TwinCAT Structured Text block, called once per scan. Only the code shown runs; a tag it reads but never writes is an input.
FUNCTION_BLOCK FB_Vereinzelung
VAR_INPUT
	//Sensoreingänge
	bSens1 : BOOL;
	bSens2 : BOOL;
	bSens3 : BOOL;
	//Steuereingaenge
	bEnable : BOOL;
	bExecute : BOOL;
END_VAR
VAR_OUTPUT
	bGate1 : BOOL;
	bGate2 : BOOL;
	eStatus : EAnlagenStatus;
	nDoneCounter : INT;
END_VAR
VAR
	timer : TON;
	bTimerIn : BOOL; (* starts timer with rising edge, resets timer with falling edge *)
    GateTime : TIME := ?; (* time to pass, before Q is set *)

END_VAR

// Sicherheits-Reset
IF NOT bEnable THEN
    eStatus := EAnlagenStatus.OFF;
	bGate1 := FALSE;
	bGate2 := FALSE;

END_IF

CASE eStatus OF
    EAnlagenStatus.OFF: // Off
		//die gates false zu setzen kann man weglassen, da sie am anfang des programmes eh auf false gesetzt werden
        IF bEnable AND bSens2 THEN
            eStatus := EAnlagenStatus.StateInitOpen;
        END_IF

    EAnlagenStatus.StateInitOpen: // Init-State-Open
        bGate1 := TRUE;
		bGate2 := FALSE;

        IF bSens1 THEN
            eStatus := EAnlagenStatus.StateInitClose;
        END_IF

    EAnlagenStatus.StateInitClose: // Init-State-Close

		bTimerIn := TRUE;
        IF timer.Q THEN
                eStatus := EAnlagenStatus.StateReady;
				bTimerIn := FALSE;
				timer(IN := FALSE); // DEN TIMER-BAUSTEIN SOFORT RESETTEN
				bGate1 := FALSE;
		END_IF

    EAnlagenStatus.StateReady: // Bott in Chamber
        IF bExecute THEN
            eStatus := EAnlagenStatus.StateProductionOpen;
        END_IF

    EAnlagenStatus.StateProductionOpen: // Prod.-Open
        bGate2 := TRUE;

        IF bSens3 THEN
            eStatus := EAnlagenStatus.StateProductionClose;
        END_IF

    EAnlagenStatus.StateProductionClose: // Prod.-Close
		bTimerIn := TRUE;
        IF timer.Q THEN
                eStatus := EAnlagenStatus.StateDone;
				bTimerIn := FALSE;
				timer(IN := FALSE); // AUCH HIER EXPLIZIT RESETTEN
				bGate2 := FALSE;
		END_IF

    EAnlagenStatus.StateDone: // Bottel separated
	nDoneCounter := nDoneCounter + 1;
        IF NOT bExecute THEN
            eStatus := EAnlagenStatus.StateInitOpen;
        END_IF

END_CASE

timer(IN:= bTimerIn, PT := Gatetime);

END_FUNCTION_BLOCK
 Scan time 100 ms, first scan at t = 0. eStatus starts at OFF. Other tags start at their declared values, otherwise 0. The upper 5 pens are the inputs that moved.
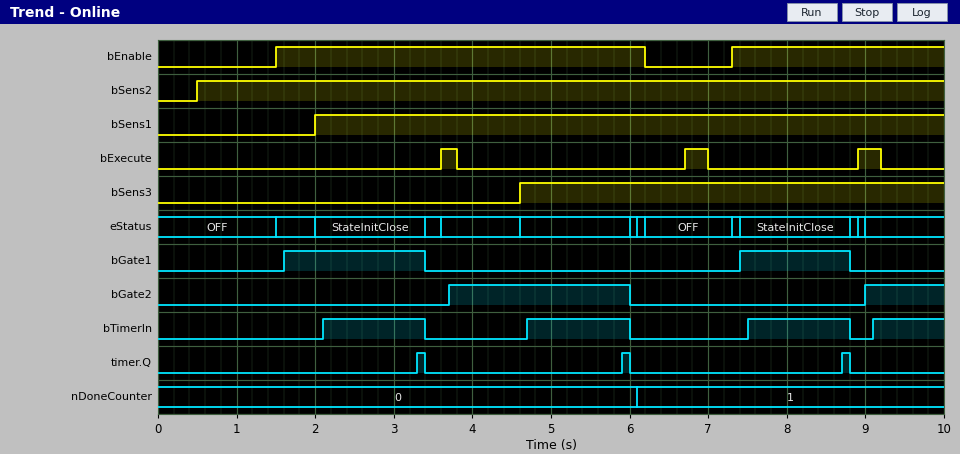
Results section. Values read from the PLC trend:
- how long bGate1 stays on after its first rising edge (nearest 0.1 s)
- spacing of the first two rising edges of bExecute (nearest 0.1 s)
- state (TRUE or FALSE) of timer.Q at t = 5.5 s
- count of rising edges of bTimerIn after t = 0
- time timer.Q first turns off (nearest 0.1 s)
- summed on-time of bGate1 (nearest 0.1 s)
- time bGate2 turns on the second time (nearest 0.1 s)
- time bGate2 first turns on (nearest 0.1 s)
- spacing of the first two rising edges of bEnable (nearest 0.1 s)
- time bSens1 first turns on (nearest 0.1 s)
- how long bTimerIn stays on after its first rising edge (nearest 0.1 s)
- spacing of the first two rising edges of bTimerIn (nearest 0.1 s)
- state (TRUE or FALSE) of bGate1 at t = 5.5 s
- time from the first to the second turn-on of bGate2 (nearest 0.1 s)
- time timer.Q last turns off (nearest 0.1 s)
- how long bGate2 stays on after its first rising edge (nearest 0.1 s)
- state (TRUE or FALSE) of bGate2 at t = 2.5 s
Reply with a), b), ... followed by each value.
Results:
a) 1.8 s
b) 3.1 s
c) FALSE
d) 4
e) 3.4 s
f) 3.2 s
g) 9.0 s
h) 3.7 s
i) 5.8 s
j) 2.0 s
k) 1.3 s
l) 2.6 s
m) FALSE
n) 5.3 s
o) 8.8 s
p) 2.3 s
q) FALSE
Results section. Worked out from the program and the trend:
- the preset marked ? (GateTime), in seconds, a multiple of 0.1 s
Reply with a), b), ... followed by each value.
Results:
a) 1.2 s
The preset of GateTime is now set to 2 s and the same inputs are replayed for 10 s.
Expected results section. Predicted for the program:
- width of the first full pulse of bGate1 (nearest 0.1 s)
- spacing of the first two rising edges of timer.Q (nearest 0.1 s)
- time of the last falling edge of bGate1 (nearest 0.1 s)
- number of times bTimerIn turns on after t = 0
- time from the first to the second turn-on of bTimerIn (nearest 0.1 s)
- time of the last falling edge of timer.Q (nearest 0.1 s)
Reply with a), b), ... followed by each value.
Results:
a) 2.6 s
b) 5.4 s
c) 9.6 s
d) 2
e) 5.4 s
f) 9.6 s
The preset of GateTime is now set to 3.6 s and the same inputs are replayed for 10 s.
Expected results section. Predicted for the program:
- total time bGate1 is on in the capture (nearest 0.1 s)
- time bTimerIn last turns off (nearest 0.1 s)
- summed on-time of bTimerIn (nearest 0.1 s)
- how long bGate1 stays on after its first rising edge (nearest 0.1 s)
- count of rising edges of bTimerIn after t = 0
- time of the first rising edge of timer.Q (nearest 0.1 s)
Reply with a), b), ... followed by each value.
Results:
a) 6.8 s
b) 5.8 s
c) 6.2 s
d) 4.2 s
e) 2
f) 5.7 s
